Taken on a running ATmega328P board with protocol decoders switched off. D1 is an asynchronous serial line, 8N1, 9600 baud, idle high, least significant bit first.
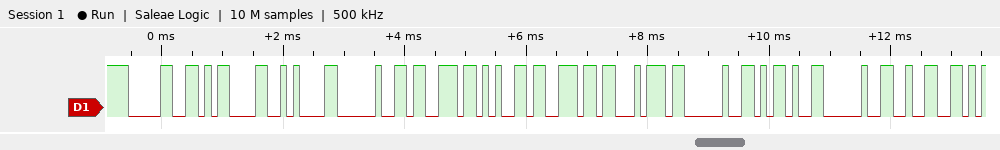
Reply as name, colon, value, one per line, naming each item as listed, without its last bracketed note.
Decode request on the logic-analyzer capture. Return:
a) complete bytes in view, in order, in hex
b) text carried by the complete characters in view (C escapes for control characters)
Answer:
complete bytes in view, in order, in hex: 30 0D 0A 20 73 65 6E 74 20 2D 20 32
text carried by the complete characters in view: "0\r\n sent - 2"
